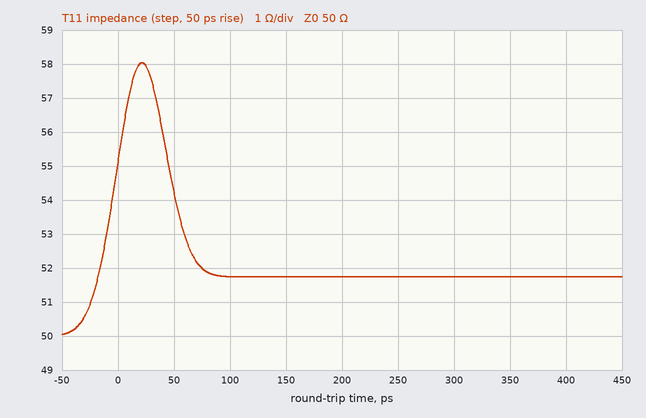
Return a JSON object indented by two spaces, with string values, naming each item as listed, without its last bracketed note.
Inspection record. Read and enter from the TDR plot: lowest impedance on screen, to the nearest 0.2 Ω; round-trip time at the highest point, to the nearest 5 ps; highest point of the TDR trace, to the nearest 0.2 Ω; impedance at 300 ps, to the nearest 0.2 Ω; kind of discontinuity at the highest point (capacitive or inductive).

{
  "lowest impedance on screen, to the nearest 0.2 Ω": "50.0 Ω",
  "round-trip time at the highest point, to the nearest 5 ps": "20 ps",
  "highest point of the TDR trace, to the nearest 0.2 Ω": "58.0 Ω",
  "impedance at 300 ps, to the nearest 0.2 Ω": "51.8 Ω",
  "kind of discontinuity at the highest point": "inductive"
}
